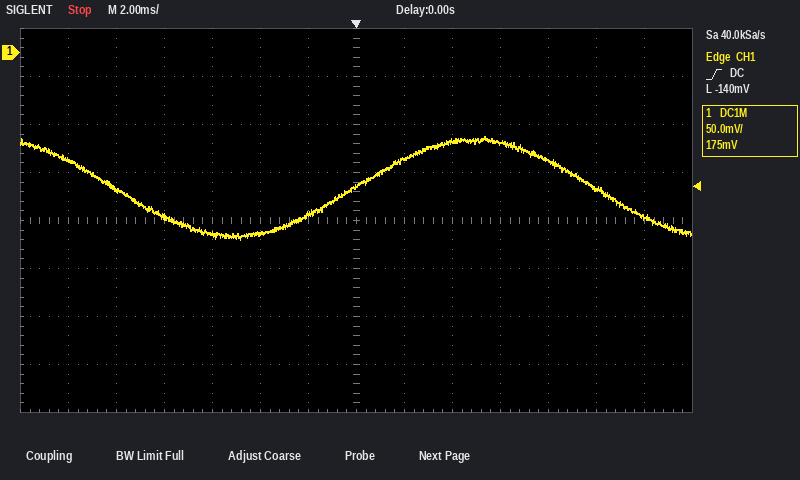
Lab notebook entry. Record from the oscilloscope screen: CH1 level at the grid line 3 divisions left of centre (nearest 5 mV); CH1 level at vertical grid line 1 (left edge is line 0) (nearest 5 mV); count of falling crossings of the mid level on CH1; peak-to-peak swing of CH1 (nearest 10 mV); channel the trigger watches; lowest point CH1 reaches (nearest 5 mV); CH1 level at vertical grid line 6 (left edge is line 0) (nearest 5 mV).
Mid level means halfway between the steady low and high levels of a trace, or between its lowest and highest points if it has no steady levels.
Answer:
-190 mV
-110 mV
2
110 mV
CH1
-195 mV
-170 mV
